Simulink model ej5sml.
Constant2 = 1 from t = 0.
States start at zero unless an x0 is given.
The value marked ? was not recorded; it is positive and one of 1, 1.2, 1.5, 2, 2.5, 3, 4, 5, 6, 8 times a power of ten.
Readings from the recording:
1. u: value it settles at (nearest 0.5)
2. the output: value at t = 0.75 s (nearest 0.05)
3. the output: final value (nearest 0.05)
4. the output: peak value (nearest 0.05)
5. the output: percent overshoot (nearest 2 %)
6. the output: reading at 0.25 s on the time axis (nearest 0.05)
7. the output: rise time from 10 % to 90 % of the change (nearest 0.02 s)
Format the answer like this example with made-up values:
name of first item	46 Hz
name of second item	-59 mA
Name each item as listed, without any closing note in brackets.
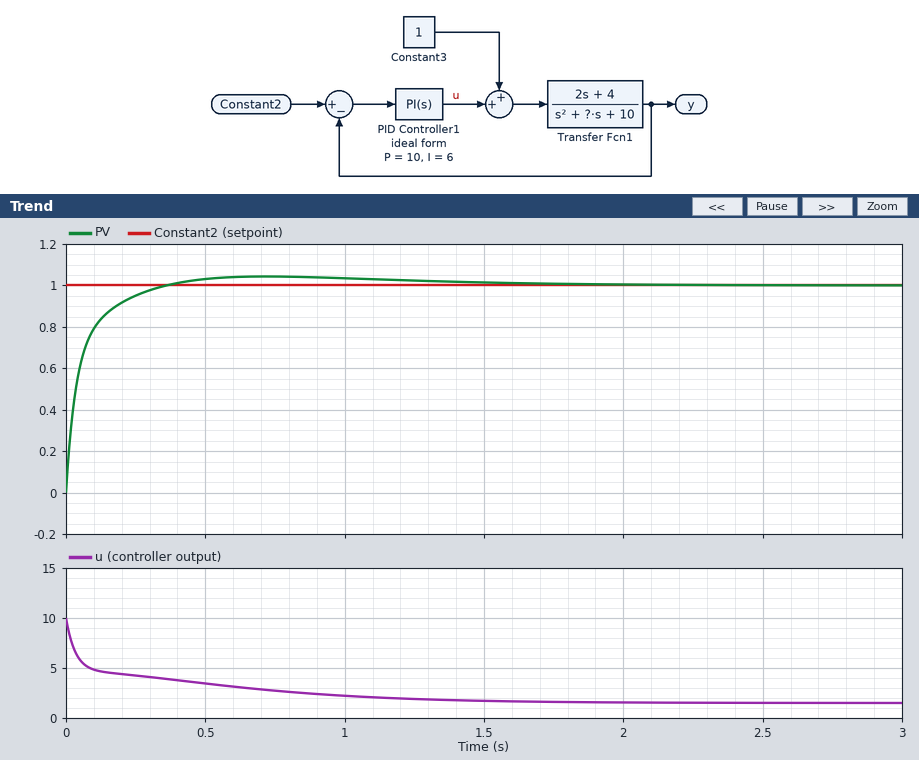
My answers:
u: value it settles at	1.5
the output: value at t = 0.75 s	1.05
the output: final value	1.00
the output: peak value	1.05
the output: percent overshoot	4 %
the output: reading at 0.25 s on the time axis	0.95
the output: rise time from 10 % to 90 % of the change	0.18 s
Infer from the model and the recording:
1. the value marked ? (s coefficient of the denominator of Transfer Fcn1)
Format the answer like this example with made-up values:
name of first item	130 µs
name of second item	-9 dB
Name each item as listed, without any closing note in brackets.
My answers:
the value marked ?	15
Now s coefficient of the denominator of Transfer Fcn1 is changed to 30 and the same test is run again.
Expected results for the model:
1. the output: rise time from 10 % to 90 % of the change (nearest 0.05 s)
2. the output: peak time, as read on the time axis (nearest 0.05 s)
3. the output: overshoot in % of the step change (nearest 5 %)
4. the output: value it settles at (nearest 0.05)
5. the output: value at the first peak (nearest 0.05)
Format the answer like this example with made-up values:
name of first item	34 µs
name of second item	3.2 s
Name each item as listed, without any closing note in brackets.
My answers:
the output: rise time from 10 % to 90 % of the change	0.35 s
the output: peak time, as read on the time axis	1.00 s
the output: overshoot in % of the step change	10 %
the output: value it settles at	1.00
the output: value at the first peak	1.10
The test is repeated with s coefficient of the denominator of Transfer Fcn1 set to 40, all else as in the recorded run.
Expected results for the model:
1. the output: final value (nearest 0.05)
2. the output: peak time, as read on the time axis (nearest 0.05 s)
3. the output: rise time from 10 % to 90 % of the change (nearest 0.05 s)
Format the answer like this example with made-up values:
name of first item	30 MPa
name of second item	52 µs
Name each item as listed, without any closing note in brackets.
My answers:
the output: final value	1.00
the output: peak time, as read on the time axis	1.10 s
the output: rise time from 10 % to 90 % of the change	0.40 s
